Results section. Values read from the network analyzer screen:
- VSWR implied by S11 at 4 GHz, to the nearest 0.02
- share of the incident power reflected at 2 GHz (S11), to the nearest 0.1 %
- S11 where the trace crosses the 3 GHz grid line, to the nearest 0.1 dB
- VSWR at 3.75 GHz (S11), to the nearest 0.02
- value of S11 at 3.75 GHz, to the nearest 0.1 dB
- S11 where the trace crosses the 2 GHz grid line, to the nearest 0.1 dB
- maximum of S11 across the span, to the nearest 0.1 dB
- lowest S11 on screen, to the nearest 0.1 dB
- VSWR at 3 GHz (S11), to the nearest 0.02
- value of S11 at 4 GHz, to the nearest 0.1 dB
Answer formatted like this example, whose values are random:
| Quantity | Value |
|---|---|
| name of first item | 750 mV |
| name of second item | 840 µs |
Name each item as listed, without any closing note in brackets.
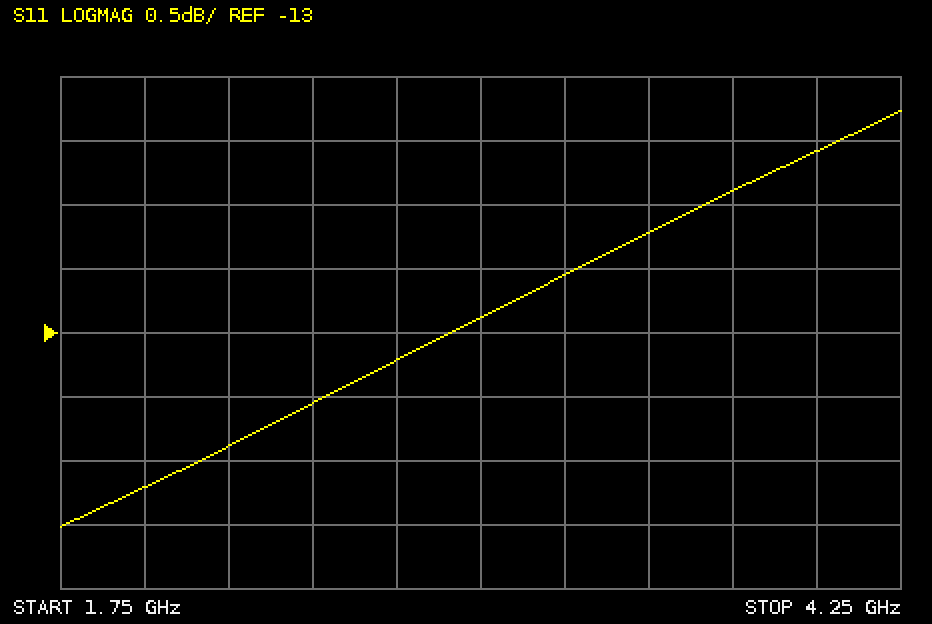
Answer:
| Quantity | Value |
|---|---|
| VSWR implied by S11 at 4 GHz, to the nearest 0.02 | 1.72 |
| share of the incident power reflected at 2 GHz (S11), to the nearest 0.1 % | 3.8 % |
| S11 where the trace crosses the 3 GHz grid line, to the nearest 0.1 dB | -12.9 dB |
| VSWR at 3.75 GHz (S11), to the nearest 0.02 | 1.68 |
| value of S11 at 3.75 GHz, to the nearest 0.1 dB | -11.9 dB |
| S11 where the trace crosses the 2 GHz grid line, to the nearest 0.1 dB | -14.2 dB |
| maximum of S11 across the span, to the nearest 0.1 dB | -11.3 dB |
| lowest S11 on screen, to the nearest 0.1 dB | -14.5 dB |
| VSWR at 3 GHz (S11), to the nearest 0.02 | 1.58 |
| value of S11 at 4 GHz, to the nearest 0.1 dB | -11.6 dB |
